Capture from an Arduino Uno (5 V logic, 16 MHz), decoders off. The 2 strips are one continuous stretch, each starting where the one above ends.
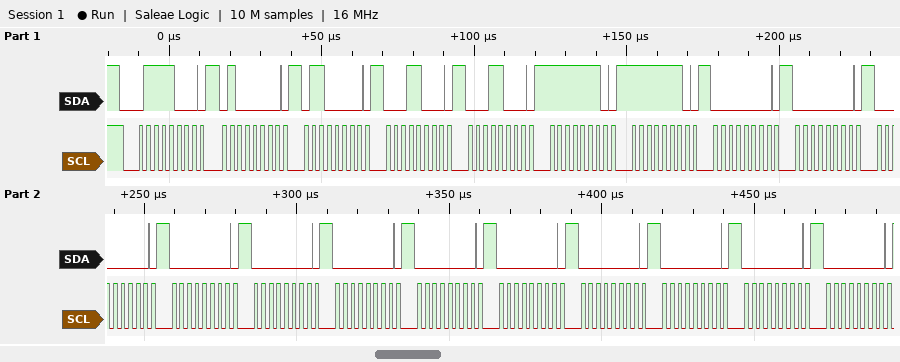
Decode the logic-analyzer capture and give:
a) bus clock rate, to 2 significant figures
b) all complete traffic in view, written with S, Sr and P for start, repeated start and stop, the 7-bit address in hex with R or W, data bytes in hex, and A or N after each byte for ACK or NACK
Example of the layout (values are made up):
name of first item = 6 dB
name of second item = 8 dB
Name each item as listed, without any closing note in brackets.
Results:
bus clock rate, to 2 significant figures = 400 kHz
all complete traffic in view, written with S, Sr and P for start, repeated start and stop, the 7-bit address in hex with R or W, data bytes in hex, and A or N after each byte for ACK or NACK = S 3CW A 40 A 60 A 18 A 18 A FE A FE A 00 A 00 A 00 A 00 A 00 A 00 A 00 A 00 A 00 A 00 A 00 A 00 A
